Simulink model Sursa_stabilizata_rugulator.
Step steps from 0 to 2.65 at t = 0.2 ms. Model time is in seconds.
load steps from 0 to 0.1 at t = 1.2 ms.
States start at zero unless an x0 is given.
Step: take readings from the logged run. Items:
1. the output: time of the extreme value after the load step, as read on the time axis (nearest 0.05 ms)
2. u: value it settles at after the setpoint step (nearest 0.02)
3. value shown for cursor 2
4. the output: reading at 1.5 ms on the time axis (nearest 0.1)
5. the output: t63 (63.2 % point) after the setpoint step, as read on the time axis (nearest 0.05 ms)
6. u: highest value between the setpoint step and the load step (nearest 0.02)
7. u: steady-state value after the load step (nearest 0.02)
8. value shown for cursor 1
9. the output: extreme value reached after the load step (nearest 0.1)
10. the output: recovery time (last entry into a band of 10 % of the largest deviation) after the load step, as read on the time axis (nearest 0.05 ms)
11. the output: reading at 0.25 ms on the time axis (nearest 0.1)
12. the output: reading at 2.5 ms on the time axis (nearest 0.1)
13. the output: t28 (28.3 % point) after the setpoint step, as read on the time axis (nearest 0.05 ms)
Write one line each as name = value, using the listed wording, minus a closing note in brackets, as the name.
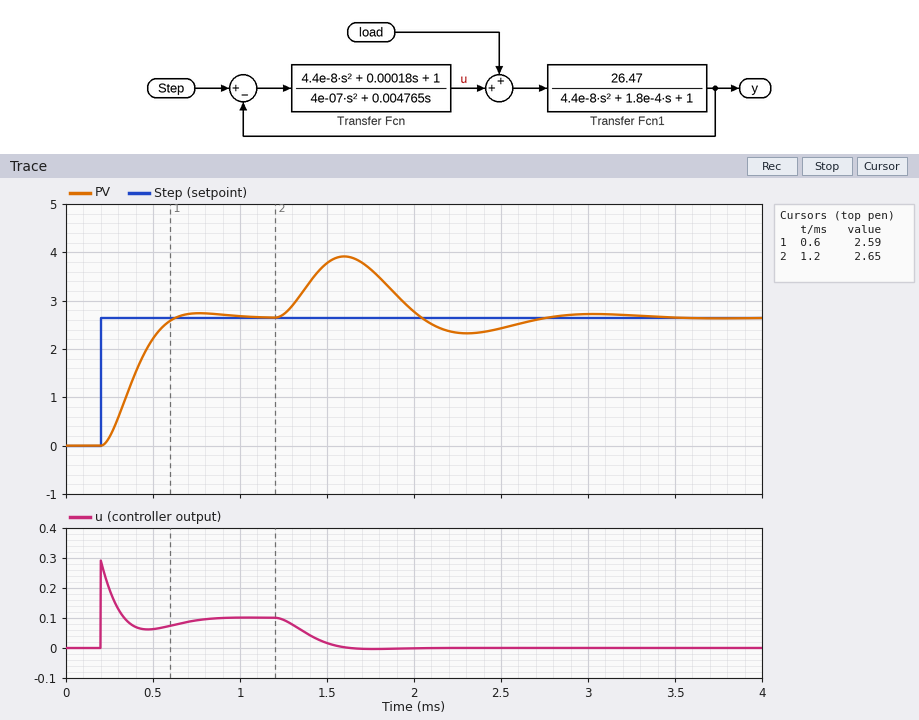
the output: time of the extreme value after the load step, as read on the time axis = 1.60 ms
u: value it settles at after the setpoint step = 0.10
value shown for cursor 2 = 2.65
the output: reading at 1.5 ms on the time axis = 3.8
the output: t63 (63.2 % point) after the setpoint step, as read on the time axis = 0.40 ms
u: highest value between the setpoint step and the load step = 0.28
u: steady-state value after the load step = 0.00
value shown for cursor 1 = 2.59
the output: extreme value reached after the load step = 3.9
the output: recovery time (last entry into a band of 10 % of the largest deviation) after the load step, as read on the time axis = 2.60 ms
the output: reading at 0.25 ms on the time axis = 0.2
the output: reading at 2.5 ms on the time axis = 2.4
the output: t28 (28.3 % point) after the setpoint step, as read on the time axis = 0.30 ms
